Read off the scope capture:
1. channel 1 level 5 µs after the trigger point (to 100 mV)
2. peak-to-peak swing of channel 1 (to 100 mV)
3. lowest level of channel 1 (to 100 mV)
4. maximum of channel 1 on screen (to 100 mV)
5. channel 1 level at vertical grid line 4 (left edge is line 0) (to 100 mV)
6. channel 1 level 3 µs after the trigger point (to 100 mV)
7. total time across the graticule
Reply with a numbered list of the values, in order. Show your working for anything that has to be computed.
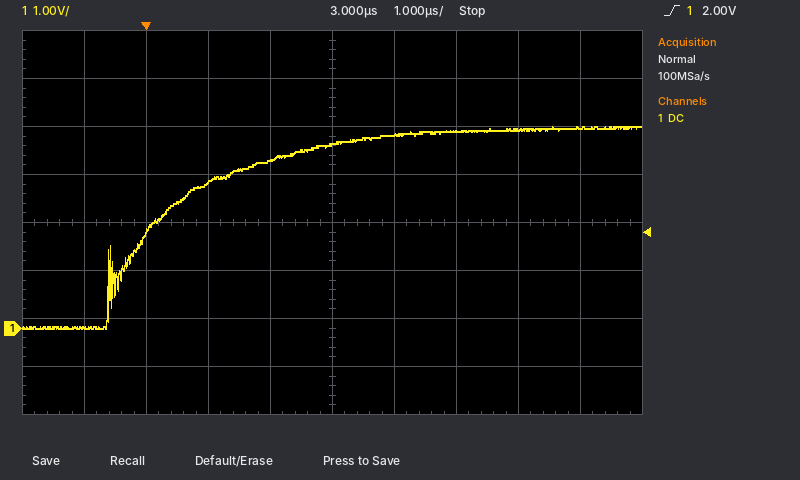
1. 4.1 V
2. 4.2 V − (0.0 V) = 4.2 V
3. 0.0 V
4. 4.2 V
5. 3.5 V
6. 3.8 V
7. 10 µs
